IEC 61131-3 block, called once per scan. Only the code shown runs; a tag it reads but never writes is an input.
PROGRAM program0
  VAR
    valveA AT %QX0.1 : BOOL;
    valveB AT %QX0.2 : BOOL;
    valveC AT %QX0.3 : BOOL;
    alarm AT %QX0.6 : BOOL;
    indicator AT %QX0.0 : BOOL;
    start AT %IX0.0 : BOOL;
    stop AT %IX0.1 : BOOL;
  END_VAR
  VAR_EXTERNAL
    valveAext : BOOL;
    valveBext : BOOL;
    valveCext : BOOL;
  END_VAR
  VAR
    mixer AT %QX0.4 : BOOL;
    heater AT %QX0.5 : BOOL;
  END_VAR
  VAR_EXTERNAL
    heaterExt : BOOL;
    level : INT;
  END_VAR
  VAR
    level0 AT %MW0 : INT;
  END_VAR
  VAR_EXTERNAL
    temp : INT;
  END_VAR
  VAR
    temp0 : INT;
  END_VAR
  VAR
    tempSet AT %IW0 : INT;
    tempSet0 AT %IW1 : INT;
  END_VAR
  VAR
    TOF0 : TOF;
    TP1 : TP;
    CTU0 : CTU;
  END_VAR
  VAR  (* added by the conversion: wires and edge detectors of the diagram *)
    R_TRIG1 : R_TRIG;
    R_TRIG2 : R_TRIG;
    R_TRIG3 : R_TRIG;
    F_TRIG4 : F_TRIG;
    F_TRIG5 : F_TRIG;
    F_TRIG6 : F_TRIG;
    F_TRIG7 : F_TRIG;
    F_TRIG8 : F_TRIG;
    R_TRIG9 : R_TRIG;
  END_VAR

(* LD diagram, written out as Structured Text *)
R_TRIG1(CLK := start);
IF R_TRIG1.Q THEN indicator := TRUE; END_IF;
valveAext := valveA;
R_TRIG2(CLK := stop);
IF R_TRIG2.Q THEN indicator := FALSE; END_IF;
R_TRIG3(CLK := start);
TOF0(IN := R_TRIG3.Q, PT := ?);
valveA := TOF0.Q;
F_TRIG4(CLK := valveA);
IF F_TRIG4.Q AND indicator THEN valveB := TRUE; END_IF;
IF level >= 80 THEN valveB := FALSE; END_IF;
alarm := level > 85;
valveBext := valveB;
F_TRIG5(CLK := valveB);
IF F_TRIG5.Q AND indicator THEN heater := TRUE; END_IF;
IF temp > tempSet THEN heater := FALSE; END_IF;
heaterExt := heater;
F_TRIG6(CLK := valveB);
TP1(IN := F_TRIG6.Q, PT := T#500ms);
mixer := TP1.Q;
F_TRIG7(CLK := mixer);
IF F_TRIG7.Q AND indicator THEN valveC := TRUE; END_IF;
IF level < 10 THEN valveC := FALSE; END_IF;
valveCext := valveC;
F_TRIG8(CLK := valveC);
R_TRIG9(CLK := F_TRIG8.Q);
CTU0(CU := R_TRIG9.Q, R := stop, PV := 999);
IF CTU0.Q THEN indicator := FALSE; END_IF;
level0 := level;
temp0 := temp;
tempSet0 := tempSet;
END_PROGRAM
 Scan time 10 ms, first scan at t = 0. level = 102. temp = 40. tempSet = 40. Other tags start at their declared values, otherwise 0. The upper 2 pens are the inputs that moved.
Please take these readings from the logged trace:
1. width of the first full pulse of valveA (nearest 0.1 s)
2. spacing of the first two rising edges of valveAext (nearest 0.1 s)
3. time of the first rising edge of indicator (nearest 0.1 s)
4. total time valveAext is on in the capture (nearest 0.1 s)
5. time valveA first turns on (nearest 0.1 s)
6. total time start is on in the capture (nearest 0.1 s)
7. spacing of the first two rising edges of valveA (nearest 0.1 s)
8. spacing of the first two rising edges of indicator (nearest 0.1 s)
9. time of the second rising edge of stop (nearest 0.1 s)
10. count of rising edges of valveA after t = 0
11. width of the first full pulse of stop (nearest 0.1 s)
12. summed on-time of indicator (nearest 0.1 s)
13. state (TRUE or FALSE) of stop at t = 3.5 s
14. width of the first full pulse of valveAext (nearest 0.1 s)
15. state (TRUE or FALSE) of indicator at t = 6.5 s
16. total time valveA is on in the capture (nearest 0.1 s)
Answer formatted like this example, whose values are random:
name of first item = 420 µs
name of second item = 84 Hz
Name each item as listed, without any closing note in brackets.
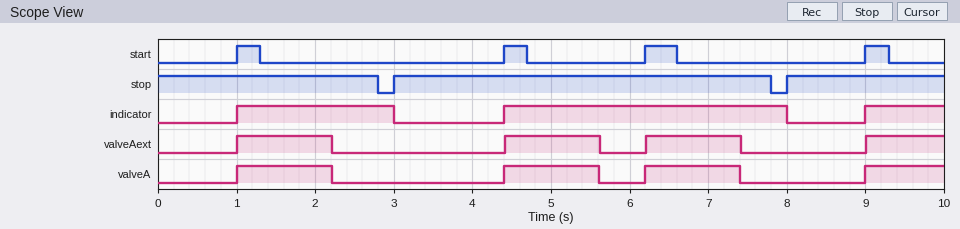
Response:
width of the first full pulse of valveA = 1.2 s
spacing of the first two rising edges of valveAext = 3.4 s
time of the first rising edge of indicator = 1.0 s
total time valveAext is on in the capture = 4.6 s
time valveA first turns on = 1.0 s
total time start is on in the capture = 1.3 s
spacing of the first two rising edges of valveA = 3.4 s
spacing of the first two rising edges of indicator = 3.4 s
time of the second rising edge of stop = 8.0 s
count of rising edges of valveA after t = 0 = 4
width of the first full pulse of stop = 4.8 s
summed on-time of indicator = 6.6 s
state (TRUE or FALSE) of stop at t = 3.5 s = TRUE
width of the first full pulse of valveAext = 1.2 s
state (TRUE or FALSE) of indicator at t = 6.5 s = TRUE
total time valveA is on in the capture = 4.6 s
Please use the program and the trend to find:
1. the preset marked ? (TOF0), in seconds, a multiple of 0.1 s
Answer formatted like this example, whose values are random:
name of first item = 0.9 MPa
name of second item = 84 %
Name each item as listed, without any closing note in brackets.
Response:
the preset marked ? (TOF0), in seconds, a multiple of 0.1 s = 1.2 s
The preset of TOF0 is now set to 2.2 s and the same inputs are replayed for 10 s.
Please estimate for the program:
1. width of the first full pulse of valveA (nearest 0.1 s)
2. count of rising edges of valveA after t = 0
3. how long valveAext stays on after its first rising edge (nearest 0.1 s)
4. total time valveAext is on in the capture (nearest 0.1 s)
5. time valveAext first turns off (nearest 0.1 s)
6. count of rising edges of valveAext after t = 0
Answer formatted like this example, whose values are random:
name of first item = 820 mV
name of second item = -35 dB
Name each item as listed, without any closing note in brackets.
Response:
width of the first full pulse of valveA = 2.2 s
count of rising edges of valveA after t = 0 = 3
how long valveAext stays on after its first rising edge = 2.2 s
total time valveAext is on in the capture = 7.2 s
time valveAext first turns off = 3.2 s
count of rising edges of valveAext after t = 0 = 3
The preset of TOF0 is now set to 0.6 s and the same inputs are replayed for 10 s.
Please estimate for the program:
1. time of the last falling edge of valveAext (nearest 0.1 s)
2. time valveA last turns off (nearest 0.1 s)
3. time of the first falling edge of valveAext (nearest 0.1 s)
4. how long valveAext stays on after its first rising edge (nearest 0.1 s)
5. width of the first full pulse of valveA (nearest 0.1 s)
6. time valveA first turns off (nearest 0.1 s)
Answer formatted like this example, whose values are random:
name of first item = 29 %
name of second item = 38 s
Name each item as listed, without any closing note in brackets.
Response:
time of the last falling edge of valveAext = 9.6 s
time valveA last turns off = 9.6 s
time of the first falling edge of valveAext = 1.6 s
how long valveAext stays on after its first rising edge = 0.6 s
width of the first full pulse of valveA = 0.6 s
time valveA first turns off = 1.6 s
